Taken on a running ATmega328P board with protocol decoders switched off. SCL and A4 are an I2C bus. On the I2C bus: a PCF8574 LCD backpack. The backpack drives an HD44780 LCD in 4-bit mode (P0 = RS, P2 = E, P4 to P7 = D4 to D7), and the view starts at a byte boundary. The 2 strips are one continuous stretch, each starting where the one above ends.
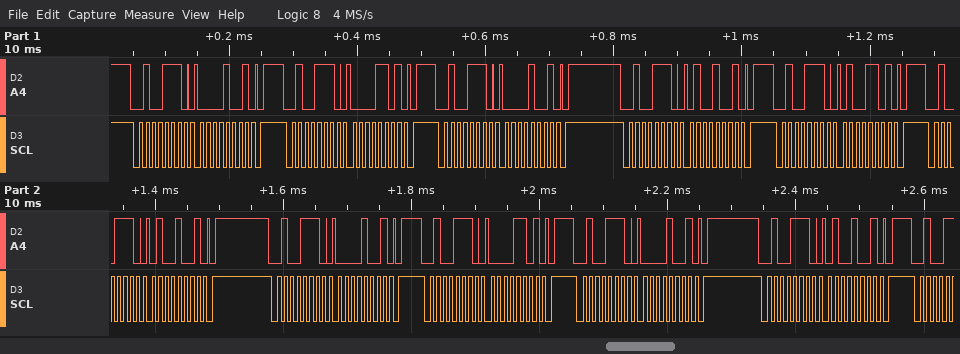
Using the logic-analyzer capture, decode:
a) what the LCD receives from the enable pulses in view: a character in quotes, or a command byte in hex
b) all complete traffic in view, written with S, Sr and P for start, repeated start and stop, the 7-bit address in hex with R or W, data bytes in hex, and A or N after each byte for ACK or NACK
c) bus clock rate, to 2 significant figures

data 0x04
S 27W A 09 A P S 27W A 0D A P S 27W A 09 A P S 27W A 49 A P S 27W A 4D A P S 27W A 49 A P S 27W A 09 A P S 27W A 0D A P S 27W A 09 A P S 27W A 49 A P
100 kHz
